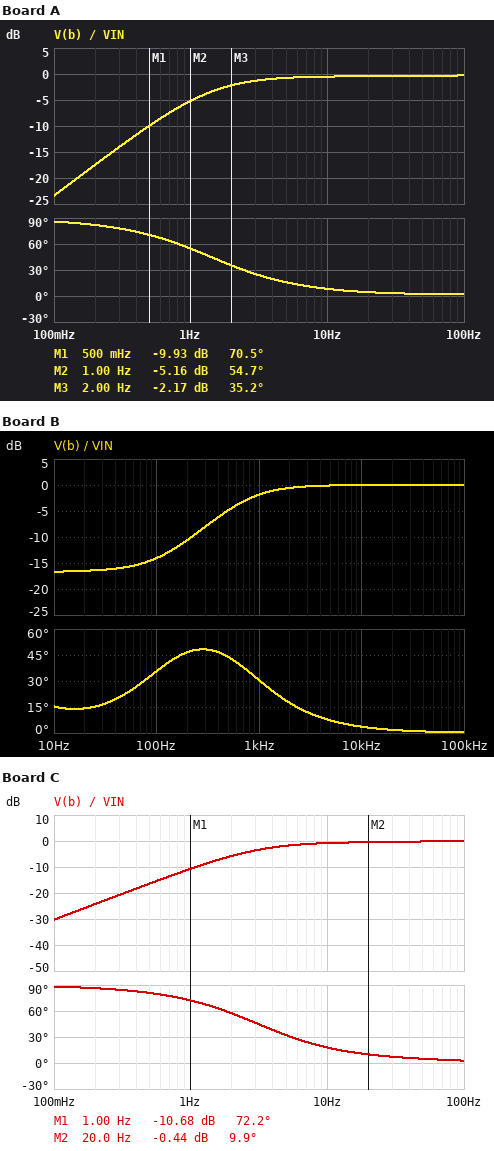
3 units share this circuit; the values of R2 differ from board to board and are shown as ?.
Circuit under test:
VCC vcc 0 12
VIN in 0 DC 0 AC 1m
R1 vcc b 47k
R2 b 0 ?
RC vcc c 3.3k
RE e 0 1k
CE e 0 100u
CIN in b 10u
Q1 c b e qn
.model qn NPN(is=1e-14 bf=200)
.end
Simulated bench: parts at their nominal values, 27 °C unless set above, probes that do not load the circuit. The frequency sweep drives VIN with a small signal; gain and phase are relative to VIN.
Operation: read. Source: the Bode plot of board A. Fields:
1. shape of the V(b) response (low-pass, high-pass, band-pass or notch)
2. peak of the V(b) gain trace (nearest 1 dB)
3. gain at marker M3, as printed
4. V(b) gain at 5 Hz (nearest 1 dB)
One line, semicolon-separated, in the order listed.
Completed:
high-pass; 0 dB; -2.17 dB; -1 dB
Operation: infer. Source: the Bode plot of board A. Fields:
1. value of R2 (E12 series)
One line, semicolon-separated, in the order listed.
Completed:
15 kΩ
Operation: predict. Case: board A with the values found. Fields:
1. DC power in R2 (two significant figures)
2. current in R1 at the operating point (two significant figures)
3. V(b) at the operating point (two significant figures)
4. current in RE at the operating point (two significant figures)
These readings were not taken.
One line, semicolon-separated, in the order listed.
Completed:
520 µW; 200 µA; 2.8 V; 2.1 mA
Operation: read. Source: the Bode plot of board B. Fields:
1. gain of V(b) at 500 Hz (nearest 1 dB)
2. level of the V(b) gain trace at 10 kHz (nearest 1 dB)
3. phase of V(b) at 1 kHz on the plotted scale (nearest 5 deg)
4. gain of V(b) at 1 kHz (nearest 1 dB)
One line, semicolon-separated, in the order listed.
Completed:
-5 dB; 0 dB; 30 deg; -2 dB
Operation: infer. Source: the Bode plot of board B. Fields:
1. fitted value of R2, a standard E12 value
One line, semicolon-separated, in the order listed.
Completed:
22 kΩ
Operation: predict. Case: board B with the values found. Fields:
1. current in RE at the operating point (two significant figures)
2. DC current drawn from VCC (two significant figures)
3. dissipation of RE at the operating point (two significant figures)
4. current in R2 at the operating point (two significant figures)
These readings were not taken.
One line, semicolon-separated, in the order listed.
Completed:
2.8 mA; 2.9 mA; 7.7 mW; 160 µA
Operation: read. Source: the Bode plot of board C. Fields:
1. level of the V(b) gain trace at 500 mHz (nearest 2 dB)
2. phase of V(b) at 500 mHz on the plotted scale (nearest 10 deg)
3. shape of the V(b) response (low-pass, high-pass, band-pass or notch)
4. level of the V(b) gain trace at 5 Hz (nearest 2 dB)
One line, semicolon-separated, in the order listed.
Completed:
-16 dB; 80 deg; high-pass; -2 dB
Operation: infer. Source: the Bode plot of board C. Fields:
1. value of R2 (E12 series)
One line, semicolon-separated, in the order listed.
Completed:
5.6 kΩ
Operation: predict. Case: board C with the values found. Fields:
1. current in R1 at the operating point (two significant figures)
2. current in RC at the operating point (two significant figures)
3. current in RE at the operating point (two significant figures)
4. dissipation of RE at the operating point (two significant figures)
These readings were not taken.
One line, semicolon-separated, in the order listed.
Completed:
230 µA; 620 µA; 620 µA; 380 µW
